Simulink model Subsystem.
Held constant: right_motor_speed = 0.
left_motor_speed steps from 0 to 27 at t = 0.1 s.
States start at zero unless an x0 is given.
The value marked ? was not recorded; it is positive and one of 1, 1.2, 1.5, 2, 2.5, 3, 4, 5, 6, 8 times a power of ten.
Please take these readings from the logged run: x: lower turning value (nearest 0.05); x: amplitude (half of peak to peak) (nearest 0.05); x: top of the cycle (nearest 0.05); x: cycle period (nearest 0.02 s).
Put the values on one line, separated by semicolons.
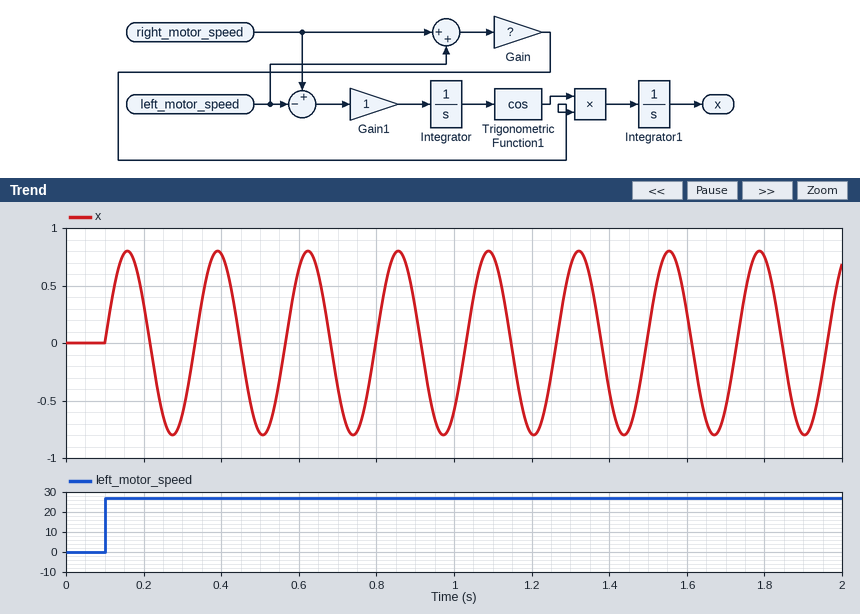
-0.80; 0.80; 0.80; 0.24 s
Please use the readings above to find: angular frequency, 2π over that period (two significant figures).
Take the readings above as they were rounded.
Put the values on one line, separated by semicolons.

26 rad/s
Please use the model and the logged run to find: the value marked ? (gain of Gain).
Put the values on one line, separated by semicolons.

0.8
